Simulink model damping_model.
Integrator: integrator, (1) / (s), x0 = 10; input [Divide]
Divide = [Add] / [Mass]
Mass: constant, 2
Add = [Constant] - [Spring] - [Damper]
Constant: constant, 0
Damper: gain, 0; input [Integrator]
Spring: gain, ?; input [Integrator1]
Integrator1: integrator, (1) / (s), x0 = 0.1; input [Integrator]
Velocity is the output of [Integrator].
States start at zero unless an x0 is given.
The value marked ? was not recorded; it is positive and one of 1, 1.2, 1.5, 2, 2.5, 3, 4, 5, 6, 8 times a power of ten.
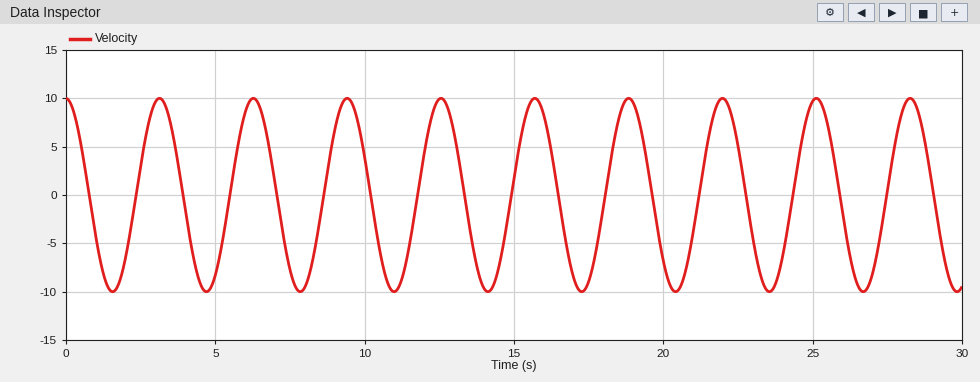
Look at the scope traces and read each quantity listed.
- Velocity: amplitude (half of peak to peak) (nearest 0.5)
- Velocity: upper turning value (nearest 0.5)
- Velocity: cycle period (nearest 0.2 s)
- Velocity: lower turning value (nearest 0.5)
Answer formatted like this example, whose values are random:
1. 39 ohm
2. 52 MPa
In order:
1. 10.0
2. 10.0
3. 3.2 s
4. -10.0
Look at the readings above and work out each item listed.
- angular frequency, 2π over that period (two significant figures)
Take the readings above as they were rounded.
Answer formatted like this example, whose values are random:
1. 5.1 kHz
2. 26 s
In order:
1. 2.0 rad/s
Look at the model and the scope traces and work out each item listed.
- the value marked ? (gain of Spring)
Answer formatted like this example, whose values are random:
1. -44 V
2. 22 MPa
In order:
1. 8
